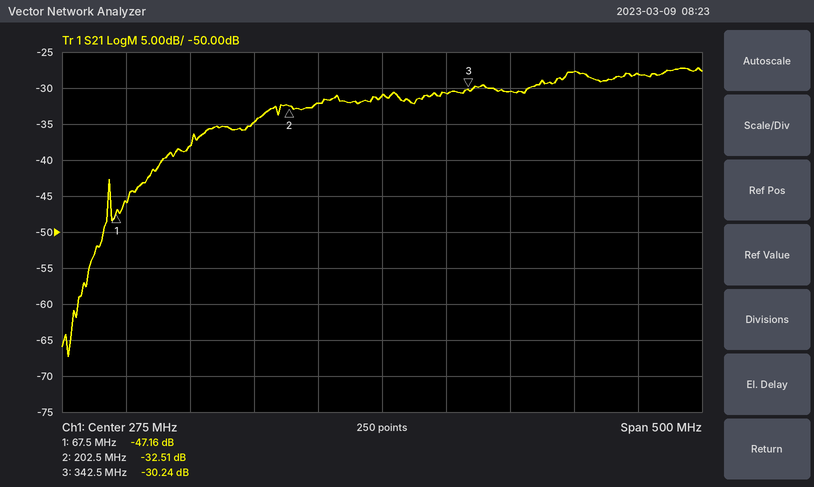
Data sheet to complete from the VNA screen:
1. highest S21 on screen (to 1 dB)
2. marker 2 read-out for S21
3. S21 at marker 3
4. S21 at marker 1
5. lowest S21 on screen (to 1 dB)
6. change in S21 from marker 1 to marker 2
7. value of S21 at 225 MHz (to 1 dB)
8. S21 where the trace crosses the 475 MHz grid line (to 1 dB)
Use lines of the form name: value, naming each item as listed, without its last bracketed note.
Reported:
highest S21 on screen: -27 dB
marker 2 read-out for S21: -32.51 dB
S21 at marker 3: -30.24 dB
S21 at marker 1: -47.16 dB
lowest S21 on screen: -67 dB
change in S21 from marker 1 to marker 2: 14.65 dB
value of S21 at 225 MHz: -32 dB
S21 where the trace crosses the 475 MHz grid line: -28 dB
